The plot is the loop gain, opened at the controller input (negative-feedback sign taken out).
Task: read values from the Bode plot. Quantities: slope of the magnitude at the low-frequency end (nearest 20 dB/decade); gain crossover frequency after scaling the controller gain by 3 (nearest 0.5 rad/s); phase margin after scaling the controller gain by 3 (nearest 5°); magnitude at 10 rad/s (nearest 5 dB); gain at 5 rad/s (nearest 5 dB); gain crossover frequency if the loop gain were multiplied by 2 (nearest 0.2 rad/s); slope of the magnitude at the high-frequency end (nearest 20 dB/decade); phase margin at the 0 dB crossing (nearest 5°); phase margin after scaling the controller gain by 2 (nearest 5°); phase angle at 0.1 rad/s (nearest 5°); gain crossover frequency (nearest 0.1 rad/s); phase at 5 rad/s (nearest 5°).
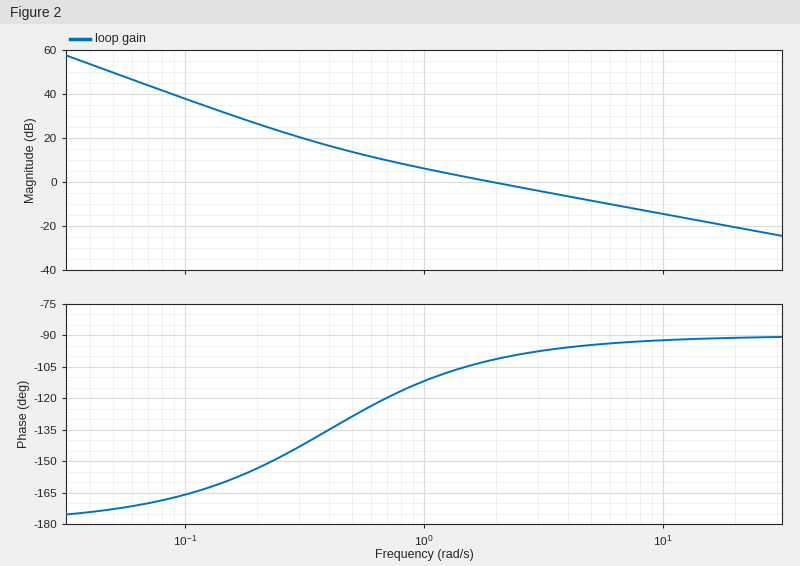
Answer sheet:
-40 dB/decade
5.5 rad/s
85°
-15 dB
-10 dB
3.8 rad/s
-20 dB/decade
80°
85°
-165°
1.9 rad/s
-95°
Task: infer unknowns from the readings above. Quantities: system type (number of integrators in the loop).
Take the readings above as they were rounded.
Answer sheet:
2
